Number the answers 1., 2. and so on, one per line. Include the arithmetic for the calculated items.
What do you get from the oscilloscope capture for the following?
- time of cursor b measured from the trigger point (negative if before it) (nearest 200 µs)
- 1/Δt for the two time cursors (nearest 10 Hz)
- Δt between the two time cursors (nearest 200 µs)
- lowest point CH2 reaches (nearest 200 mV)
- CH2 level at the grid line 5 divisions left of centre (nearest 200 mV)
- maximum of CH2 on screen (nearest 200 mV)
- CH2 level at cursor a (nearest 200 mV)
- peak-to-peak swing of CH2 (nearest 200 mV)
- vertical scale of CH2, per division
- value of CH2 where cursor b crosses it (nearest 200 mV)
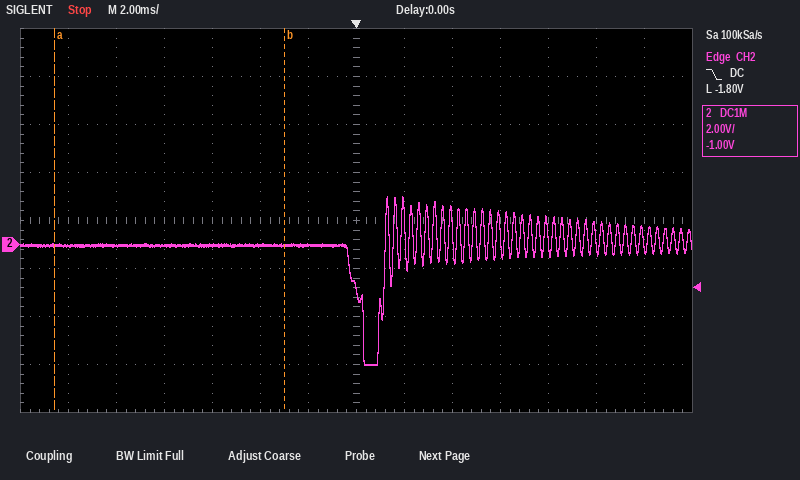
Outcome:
1. -3.0 ms
2. 1 / 9.6 ms ≈ 100 Hz
3. 9.6 ms
4. -5.0 V
5. 0.0 V
6. 2.0 V
7. 0.0 V
8. 2.0 V − (-5.0 V) = 7.0 V
9. 2 V
10. 0.0 V
